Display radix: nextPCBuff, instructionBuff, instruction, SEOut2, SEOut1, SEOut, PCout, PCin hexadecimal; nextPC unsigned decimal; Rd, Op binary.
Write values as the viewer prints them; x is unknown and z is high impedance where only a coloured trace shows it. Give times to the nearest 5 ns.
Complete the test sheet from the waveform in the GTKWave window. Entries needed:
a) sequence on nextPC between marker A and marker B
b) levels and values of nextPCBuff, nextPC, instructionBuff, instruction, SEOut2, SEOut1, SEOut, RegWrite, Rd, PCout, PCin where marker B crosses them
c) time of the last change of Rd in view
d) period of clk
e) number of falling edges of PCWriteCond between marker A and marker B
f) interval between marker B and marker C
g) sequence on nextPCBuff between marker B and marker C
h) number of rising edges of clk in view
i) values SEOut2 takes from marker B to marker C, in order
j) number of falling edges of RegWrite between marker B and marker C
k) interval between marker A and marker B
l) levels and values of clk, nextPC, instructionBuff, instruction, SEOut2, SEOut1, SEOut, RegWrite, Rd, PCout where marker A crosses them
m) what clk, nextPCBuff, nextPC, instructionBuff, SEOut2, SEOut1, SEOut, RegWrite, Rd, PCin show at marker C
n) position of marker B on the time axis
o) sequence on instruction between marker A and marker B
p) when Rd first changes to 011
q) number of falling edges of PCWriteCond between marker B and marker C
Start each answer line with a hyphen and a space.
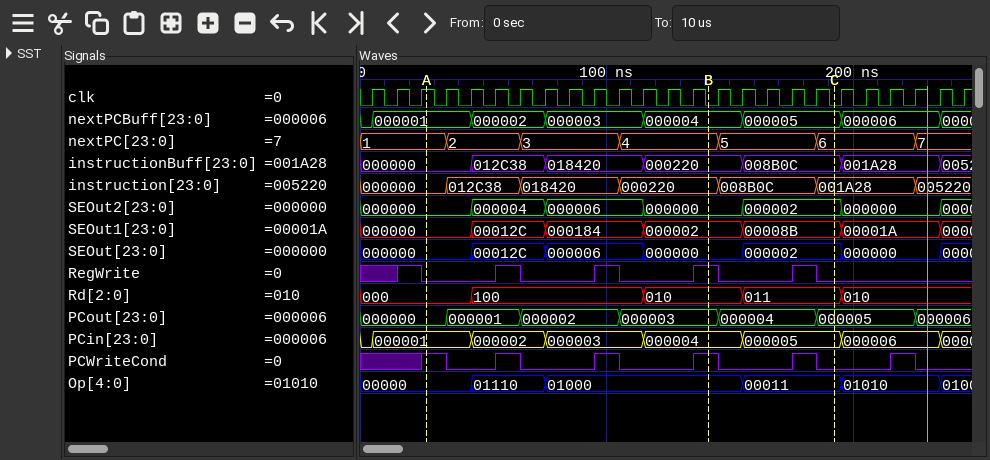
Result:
- 1, 2, 3, 4
- nextPCBuff=000004, nextPC=4, instructionBuff=000220, instruction=000220, SEOut2=000000, SEOut1=000002, SEOut=000000, RegWrite=1, Rd=010, PCout=000003, PCin=000004
- 195 ns
- 10 ns
- 3
- 50 ns
- 000004, 000005
- 25
- 000000, 000002
- 2
- 115 ns
- clk=1, nextPC=1, instructionBuff=000000, instruction=000000, SEOut2=000000, SEOut1=000000, SEOut=000000, RegWrite=0, Rd=000, PCout=000000
- clk=0, nextPCBuff=000005, nextPC=6, instructionBuff=008B0C, SEOut2=000002, SEOut1=00008B, SEOut=000002, RegWrite=0, Rd=011, PCin=000005
- 140 ns
- 000000, 012C38, 018420, 000220
- 155 ns
- 2
